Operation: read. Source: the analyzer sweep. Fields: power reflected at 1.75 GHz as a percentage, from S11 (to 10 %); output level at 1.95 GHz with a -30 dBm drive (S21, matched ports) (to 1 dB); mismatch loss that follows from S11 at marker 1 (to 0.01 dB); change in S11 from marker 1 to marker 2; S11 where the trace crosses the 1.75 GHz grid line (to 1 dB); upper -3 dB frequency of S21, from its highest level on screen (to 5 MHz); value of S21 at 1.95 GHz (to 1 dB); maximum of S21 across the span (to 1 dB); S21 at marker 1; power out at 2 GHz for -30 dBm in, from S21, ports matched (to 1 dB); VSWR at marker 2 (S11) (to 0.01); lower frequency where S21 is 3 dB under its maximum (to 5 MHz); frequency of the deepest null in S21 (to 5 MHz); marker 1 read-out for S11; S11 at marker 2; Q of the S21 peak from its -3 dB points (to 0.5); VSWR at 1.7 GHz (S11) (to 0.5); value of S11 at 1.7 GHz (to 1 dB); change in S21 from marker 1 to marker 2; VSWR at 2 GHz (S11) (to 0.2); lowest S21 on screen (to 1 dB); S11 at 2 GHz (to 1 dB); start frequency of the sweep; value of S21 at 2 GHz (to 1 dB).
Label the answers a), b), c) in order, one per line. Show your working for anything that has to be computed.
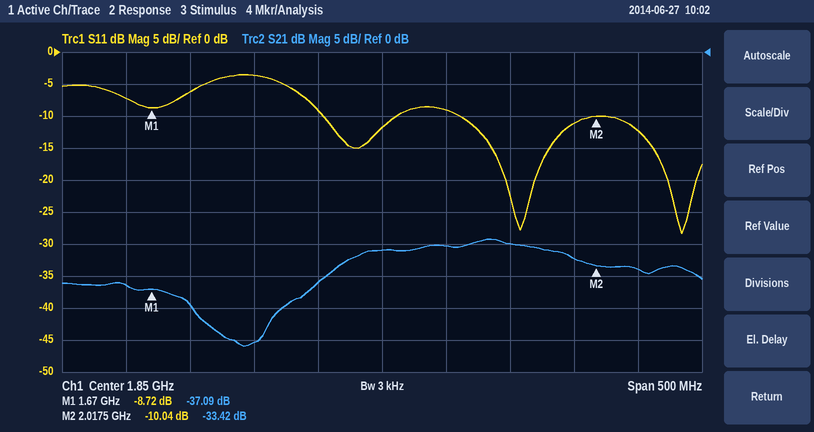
a) 10^(-4/10) ≈ 40 %
b) -30 dBm + (-30 dB) = -60 dBm
c) −10 log10(1 − 10^(-8.72/10)) ≈ 0.63 dB
d) -10.04 − (-8.72) = -1.32 dB
e) -4 dB
f) 2.000 GHz
g) -30 dB
h) -29 dB
i) -37.09 dB
j) -30 dBm + (-32 dB) = -62 dBm
k) (1 + 0.3148)/(1 − 0.3148) ≈ 1.92
l) 1.825 GHz
m) 1.740 GHz
n) -8.72 dB
o) -10.04 dB
p) 1.9125 GHz / 175 MHz ≈ 10.9, so 11.0 to the nearest 0.5
q) |Γ| = 10^(-6/20) = 0.5012; VSWR = (1 + 0.5012)/(1 − 0.5012) ≈ 3.0
r) -6 dB
s) -33.42 − (-37.09) = 3.67 dB
t) |Γ| = 10^(-11/20) = 0.2818; VSWR = (1 + 0.2818)/(1 − 0.2818) ≈ 1.8
u) -46 dB
v) -11 dB
w) 1.6 GHz
x) -32 dB
